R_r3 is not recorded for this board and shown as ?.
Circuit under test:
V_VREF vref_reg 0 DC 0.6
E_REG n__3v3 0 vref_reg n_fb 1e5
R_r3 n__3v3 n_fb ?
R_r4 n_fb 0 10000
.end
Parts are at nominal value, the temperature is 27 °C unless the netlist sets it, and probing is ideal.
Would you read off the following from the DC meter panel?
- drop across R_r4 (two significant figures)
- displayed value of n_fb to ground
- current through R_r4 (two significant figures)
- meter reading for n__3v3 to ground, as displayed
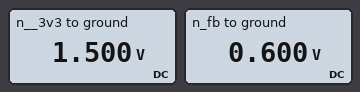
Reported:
600 mV
0.600 V
60 µA
1.500 V
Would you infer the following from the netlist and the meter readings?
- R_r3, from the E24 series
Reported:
15 kΩ
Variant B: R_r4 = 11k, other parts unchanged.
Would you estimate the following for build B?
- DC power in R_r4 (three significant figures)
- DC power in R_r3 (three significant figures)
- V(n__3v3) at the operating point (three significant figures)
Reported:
32.7 µW
44.6 µW
1.42 V
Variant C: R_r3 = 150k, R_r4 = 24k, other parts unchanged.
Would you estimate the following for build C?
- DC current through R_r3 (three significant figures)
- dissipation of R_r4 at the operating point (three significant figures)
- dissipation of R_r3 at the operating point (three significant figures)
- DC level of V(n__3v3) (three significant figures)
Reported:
25.0 µA
15.0 µW
93.7 µW
4.35 V
